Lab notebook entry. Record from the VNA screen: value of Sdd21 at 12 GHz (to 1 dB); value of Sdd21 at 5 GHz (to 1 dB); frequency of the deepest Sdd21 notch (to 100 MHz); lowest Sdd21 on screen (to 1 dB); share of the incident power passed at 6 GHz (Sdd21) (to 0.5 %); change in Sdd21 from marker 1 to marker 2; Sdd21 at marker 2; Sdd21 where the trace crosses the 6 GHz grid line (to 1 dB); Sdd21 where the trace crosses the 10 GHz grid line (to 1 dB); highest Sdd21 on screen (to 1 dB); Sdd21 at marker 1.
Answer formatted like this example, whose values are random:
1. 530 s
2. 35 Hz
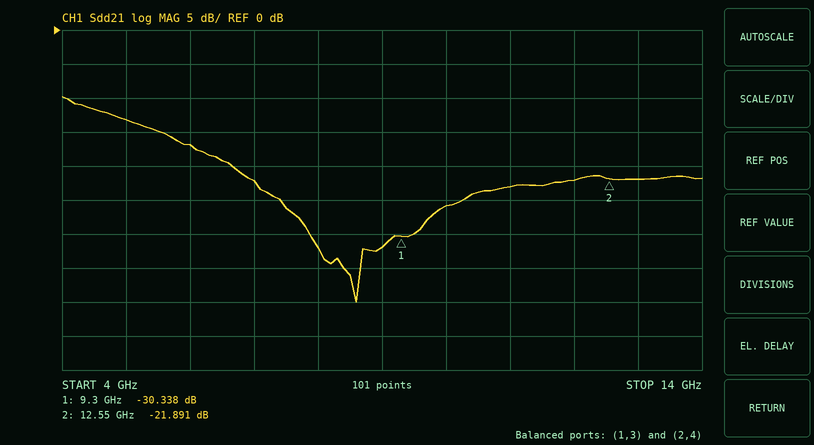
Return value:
1. -22 dB
2. -13 dB
3. 8.6 GHz
4. -40 dB
5. 2.0 %
6. 8.447 dB
7. -21.891 dB
8. -17 dB
9. -26 dB
10. -10 dB
11. -30.338 dB
